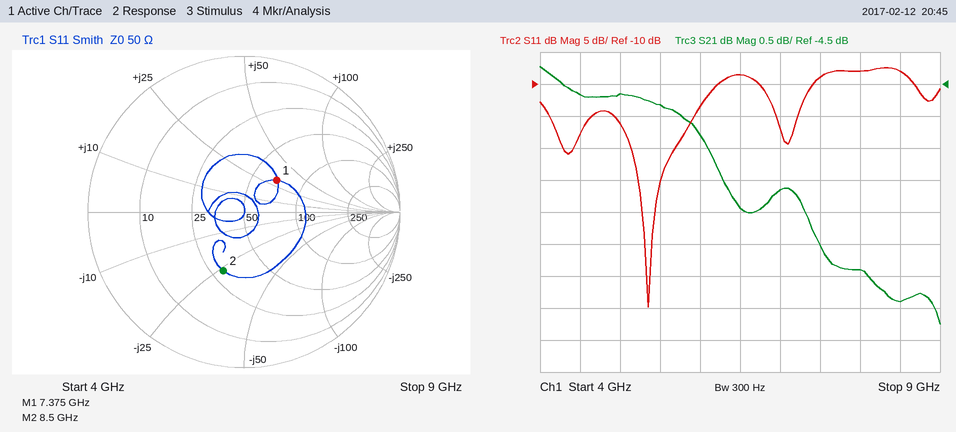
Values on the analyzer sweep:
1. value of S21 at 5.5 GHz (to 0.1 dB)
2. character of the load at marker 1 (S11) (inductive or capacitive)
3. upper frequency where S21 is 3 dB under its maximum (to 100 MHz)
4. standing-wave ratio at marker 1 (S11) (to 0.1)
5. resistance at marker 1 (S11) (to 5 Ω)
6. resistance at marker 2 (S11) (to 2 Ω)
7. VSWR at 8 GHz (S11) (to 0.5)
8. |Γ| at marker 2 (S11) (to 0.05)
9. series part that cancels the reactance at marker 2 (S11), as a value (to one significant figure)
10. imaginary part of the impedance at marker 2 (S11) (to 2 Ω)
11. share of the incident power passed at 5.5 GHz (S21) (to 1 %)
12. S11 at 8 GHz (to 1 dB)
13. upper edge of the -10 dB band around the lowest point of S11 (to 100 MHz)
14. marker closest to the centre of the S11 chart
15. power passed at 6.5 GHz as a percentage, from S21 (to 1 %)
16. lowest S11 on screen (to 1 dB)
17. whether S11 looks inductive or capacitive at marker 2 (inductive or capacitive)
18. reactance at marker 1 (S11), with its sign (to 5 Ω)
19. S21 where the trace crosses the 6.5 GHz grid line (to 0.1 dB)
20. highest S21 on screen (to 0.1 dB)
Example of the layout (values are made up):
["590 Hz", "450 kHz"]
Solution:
["-4.8 dB", "inductive", "7.6 GHz", "1.8", "70 Ω", "30 Ω", "2.5", "0.40", "500 pH", "-26 Ω", "33 %", "-8 dB", "6.2 GHz", "marker 1", "23 %", "-45 dB", "capacitive", "+30 Ω", "-6.4 dB", "-4.2 dB"]
